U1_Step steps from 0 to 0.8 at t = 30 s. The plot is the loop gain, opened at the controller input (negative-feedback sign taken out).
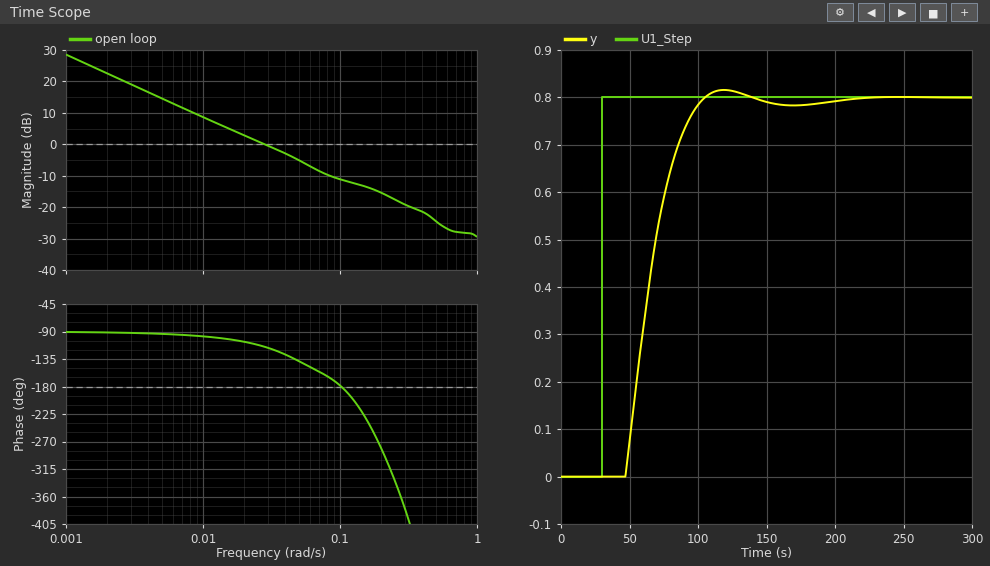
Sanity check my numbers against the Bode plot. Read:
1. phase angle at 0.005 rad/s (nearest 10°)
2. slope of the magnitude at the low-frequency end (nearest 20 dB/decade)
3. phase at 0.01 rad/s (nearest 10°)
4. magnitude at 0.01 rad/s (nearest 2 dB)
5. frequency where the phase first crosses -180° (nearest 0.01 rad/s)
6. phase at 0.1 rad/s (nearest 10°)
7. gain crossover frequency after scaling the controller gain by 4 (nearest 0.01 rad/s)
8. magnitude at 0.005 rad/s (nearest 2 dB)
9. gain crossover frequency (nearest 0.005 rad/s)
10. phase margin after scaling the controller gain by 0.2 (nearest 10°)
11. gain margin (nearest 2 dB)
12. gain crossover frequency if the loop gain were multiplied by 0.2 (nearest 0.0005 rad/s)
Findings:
-90°
-20 dB/decade
-100°
8 dB
0.10 rad/s
-180°
0.12 rad/s
14 dB
0.030 rad/s
90°
12 dB
0.0055 rad/s
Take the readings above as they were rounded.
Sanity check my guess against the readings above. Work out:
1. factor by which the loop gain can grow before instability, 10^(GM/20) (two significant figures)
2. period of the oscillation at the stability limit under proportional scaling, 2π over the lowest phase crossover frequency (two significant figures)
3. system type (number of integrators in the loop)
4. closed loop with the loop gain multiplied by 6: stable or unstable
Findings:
4.0
63 s
1
unstable
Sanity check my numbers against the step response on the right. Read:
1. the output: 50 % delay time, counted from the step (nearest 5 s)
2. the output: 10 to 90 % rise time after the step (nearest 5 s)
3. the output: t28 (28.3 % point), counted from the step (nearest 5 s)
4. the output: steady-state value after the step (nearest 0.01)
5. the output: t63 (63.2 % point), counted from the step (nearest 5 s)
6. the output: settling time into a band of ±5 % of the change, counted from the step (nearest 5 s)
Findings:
35 s
40 s
25 s
0.80
40 s
65 s
